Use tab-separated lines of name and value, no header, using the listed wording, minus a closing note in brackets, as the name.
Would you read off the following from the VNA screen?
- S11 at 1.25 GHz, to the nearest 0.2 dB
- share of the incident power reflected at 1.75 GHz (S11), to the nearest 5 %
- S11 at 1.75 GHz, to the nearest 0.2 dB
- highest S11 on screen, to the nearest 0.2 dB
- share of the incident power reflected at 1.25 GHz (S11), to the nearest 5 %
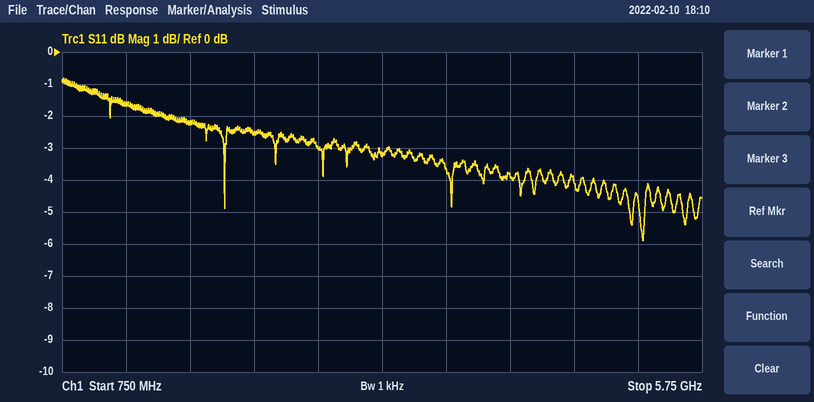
S11 at 1.25 GHz, to the nearest 0.2 dB	-1.6 dB
share of the incident power reflected at 1.75 GHz (S11), to the nearest 5 %	60 %
S11 at 1.75 GHz, to the nearest 0.2 dB	-2.2 dB
highest S11 on screen, to the nearest 0.2 dB	-0.8 dB
share of the incident power reflected at 1.25 GHz (S11), to the nearest 5 %	70 %
